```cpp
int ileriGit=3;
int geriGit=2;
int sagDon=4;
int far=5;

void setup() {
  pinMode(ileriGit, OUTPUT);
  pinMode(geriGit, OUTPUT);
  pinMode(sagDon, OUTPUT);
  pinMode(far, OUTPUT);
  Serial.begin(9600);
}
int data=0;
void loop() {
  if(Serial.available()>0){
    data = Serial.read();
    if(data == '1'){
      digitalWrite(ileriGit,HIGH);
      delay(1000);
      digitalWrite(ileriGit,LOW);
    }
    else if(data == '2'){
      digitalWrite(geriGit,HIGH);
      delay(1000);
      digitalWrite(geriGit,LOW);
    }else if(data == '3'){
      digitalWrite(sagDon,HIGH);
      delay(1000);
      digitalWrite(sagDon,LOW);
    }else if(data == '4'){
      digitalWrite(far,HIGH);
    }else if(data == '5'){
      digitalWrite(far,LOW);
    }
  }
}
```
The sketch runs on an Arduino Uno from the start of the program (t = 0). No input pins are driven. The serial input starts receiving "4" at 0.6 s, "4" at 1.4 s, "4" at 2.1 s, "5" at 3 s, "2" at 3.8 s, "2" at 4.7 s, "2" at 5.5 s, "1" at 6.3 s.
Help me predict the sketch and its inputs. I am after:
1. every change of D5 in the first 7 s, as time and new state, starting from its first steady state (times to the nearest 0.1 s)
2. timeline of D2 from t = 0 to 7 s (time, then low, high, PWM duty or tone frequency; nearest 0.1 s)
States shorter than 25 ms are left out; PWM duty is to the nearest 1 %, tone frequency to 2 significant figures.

0 s low; 0.6 s high; 3 s low
0 s low; 3.8 s high; 6.8 s low
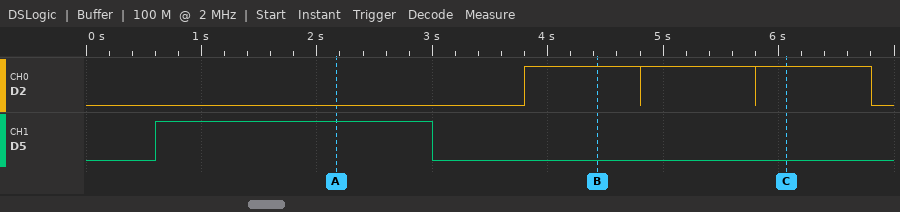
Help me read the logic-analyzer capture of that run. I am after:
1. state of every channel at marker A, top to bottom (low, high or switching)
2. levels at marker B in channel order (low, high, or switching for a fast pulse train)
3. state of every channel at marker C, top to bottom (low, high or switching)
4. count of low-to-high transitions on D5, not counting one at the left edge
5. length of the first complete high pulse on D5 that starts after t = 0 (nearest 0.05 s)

D2 low, D5 high
D2 high, D5 low
D2 high, D5 low
1
2.40 s
